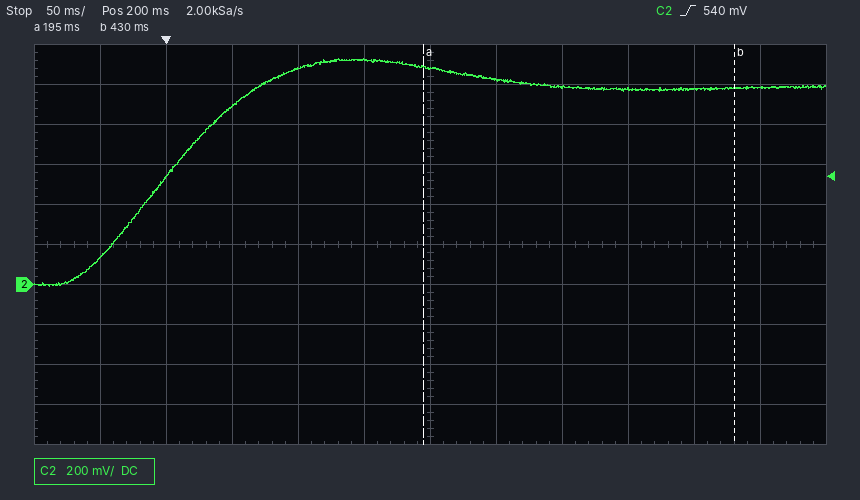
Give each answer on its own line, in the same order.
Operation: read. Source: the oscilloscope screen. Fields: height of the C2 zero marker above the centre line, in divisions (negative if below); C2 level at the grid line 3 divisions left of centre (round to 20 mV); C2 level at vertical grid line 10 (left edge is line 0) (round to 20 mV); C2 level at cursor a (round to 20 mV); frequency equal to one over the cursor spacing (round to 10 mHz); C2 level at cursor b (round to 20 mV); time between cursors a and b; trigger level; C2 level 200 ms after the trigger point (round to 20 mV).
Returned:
-1.0 div
900 mV
980 mV
1.08 V
4.26 Hz
980 mV
235 ms
540 mV
1.08 V
